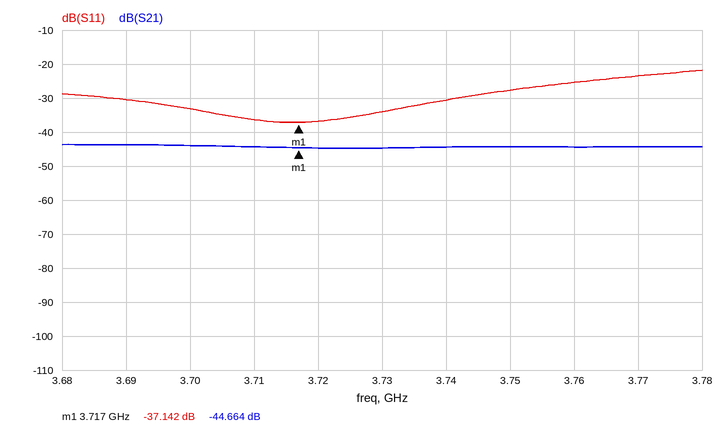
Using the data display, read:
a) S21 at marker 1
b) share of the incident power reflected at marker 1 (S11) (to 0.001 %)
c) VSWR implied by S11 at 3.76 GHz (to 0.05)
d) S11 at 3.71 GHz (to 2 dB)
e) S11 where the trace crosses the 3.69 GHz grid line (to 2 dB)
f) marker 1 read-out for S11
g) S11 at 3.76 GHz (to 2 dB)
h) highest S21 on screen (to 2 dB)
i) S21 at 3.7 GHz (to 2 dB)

-44.664 dB
0.019 %
1.10
-36 dB
-30 dB
-37.142 dB
-26 dB
-44 dB
-44 dB
